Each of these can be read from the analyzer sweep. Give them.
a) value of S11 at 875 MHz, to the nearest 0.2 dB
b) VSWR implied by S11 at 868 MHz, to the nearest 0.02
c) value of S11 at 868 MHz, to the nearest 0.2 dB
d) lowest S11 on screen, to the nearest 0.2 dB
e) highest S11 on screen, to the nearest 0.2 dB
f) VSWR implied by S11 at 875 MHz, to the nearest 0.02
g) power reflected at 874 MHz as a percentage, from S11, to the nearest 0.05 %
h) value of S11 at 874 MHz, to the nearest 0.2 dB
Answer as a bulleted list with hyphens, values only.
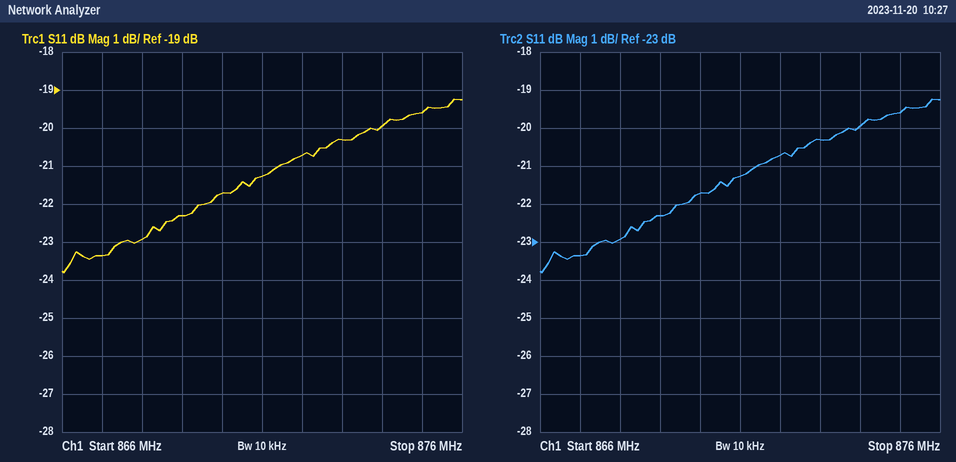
- -19.6 dB
- 1.16
- -23.0 dB
- -23.8 dB
- -19.2 dB
- 1.24
- 1.00 %
- -20.0 dB
